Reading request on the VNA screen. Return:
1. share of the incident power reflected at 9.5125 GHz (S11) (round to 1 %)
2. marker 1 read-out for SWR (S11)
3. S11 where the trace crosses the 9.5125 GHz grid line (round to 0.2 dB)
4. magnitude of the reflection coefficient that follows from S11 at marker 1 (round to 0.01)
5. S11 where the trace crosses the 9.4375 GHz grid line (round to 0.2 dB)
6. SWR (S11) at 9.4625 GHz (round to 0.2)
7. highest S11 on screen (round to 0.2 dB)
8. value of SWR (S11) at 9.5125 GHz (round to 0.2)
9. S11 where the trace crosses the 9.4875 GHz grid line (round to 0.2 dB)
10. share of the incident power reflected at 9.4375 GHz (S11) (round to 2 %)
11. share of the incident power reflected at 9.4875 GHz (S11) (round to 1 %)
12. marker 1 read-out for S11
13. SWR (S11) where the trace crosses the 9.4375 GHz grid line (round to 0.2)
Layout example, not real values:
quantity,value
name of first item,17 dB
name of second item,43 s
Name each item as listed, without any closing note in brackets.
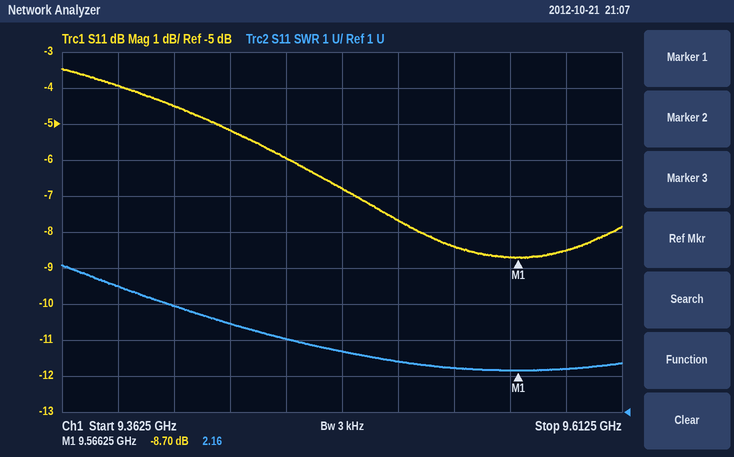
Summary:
quantity,value
share of the incident power reflected at 9.5125 GHz (S11),17 %
marker 1 read-out for SWR,2.16
S11 where the trace crosses the 9.5125 GHz grid line,-7.6 dB
magnitude of the reflection coefficient that follows from S11 at marker 1,0.37
S11 where the trace crosses the 9.4375 GHz grid line,-5.2 dB
SWR (S11) at 9.4625 GHz,3.0
highest S11 on screen,-3.4 dB
value of SWR (S11) at 9.5125 GHz,2.4
S11 where the trace crosses the 9.4875 GHz grid line,-6.8 dB
share of the incident power reflected at 9.4375 GHz (S11),30 %
share of the incident power reflected at 9.4875 GHz (S11),21 %
marker 1 read-out for S11,-8.70 dB
SWR (S11) where the trace crosses the 9.4375 GHz grid line,3.4
